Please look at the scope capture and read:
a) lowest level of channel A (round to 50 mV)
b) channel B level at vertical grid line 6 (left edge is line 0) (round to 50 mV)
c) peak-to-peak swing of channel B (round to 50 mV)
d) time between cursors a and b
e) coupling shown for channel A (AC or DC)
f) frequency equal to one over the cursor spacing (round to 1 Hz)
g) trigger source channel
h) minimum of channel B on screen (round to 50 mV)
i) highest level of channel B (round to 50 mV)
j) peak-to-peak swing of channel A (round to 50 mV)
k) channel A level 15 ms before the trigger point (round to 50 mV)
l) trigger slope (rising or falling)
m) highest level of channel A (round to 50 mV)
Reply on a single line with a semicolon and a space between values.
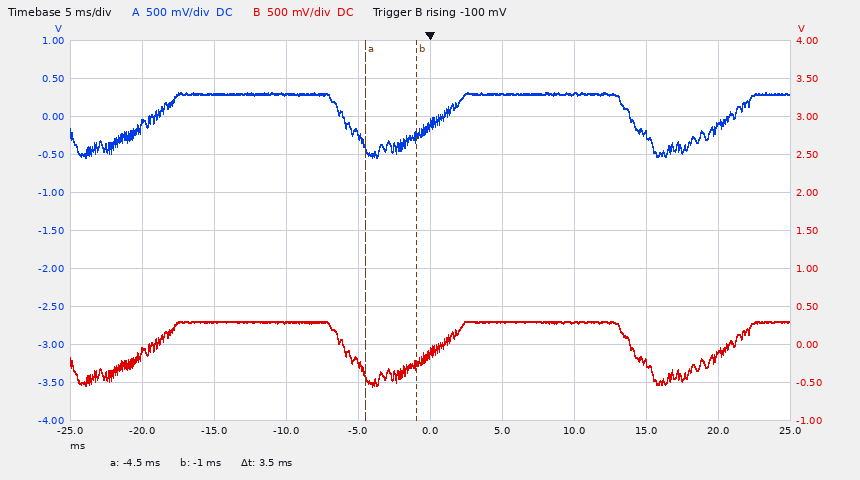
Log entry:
-550 mV; 300 mV; 850 mV; 3.5 ms; DC; 286 Hz; channel B; -550 mV; 300 mV; 850 mV; 300 mV; rising; 300 mV
